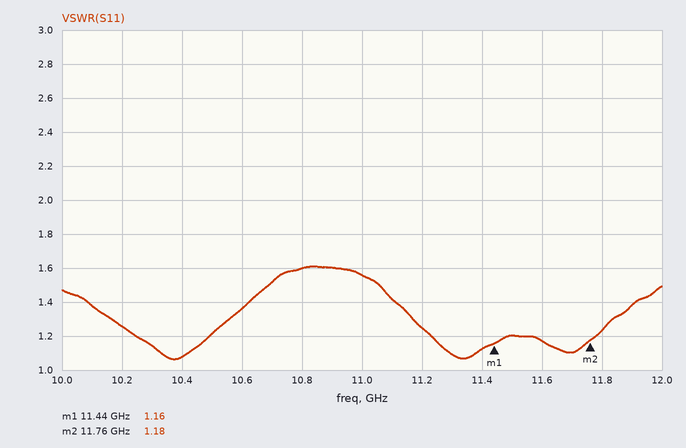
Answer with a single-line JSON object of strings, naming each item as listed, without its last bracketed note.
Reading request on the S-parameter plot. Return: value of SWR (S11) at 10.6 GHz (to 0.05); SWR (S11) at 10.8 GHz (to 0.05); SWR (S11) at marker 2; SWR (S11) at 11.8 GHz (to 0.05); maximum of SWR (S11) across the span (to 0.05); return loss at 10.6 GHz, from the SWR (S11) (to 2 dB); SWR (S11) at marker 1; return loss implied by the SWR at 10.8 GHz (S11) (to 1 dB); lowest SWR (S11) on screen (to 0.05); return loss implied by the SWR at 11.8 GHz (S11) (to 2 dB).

{"value of SWR (S11) at 10.6 GHz": "1.35", "SWR (S11) at 10.8 GHz": "1.60", "SWR (S11) at marker 2": "1.18", "SWR (S11) at 11.8 GHz": "1.25", "maximum of SWR (S11) across the span": "1.60", "return loss at 10.6 GHz, from the SWR (S11)": "16 dB", "SWR (S11) at marker 1": "1.16", "return loss implied by the SWR at 10.8 GHz (S11)": "13 dB", "lowest SWR (S11) on screen": "1.05", "return loss implied by the SWR at 11.8 GHz (S11)": "20 dB"}
